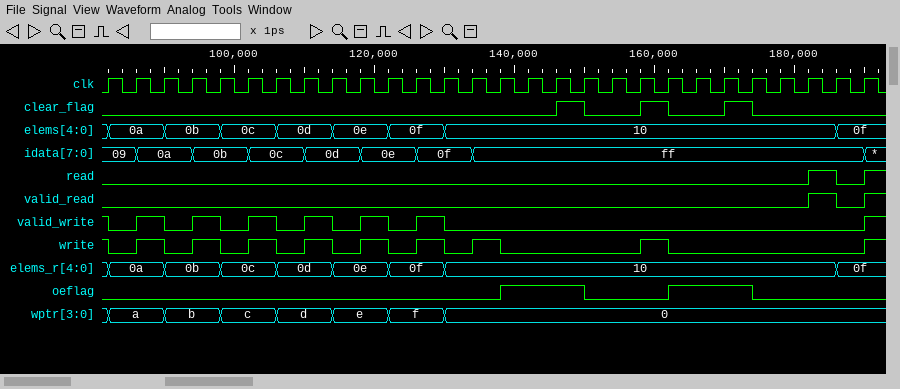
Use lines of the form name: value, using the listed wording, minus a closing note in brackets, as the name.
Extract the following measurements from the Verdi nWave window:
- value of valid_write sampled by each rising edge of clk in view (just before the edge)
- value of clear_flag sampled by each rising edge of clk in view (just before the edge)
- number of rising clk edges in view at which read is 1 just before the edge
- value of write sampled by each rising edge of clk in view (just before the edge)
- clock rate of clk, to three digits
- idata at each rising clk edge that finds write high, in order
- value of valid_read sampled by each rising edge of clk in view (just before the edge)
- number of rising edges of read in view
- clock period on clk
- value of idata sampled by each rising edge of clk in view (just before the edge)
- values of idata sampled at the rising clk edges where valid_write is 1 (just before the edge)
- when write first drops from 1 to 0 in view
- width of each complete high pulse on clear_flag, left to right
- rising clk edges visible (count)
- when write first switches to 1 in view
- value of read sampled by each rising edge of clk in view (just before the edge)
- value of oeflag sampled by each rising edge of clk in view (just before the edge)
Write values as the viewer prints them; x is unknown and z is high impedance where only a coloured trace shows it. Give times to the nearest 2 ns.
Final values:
value of valid_write sampled by each rising edge of clk in view: 1 0 1 0 1 0 1 0 1 0 1 0 1 0 0 0 0 0 0 0 0 0 0 0 0 0 0 0
value of clear_flag sampled by each rising edge of clk in view: 0 0 0 0 0 0 0 0 0 0 0 0 0 0 0 0 0 1 0 0 1 0 0 1 0 0 0 0
number of rising clk edges in view at which read is 1 just before the edge: 1
value of write sampled by each rising edge of clk in view: 1 0 1 0 1 0 1 0 1 0 1 0 1 0 1 0 0 0 0 0 1 0 0 0 0 0 0 0
clock rate of clk, to three digits: 250 MHz
idata at each rising clk edge that finds write high, in order: 09, 0a, 0b, 0c, 0d, 0e, 0f, ff, ff
value of valid_read sampled by each rising edge of clk in view: 0 0 0 0 0 0 0 0 0 0 0 0 0 0 0 0 0 0 0 0 0 0 0 0 0 0 1 0
number of rising edges of read in view: 2
clock period on clk: 4 ns
value of idata sampled by each rising edge of clk in view: 09, 09, 0a, 0a, 0b, 0b, 0c, 0c, 0d, 0d, 0e, 0e, 0f, 0f, ff, ff, ff, ff, ff, ff, ff, ff, ff, ff, ff, ff, ff, ff
values of idata sampled at the rising clk edges where valid_write is 1: 09, 0a, 0b, 0c, 0d, 0e, 0f
when write first drops from 1 to 0 in view: 82 ns
width of each complete high pulse on clear_flag, left to right: 4 ns, 4 ns, 4 ns
rising clk edges visible: 28
when write first switches to 1 in view: 86 ns
value of read sampled by each rising edge of clk in view: 0 0 0 0 0 0 0 0 0 0 0 0 0 0 0 0 0 0 0 0 0 0 0 0 0 0 1 0
value of oeflag sampled by each rising edge of clk in view: 0 0 0 0 0 0 0 0 0 0 0 0 0 0 0 1 1 1 0 0 0 1 1 1 0 0 0 0
